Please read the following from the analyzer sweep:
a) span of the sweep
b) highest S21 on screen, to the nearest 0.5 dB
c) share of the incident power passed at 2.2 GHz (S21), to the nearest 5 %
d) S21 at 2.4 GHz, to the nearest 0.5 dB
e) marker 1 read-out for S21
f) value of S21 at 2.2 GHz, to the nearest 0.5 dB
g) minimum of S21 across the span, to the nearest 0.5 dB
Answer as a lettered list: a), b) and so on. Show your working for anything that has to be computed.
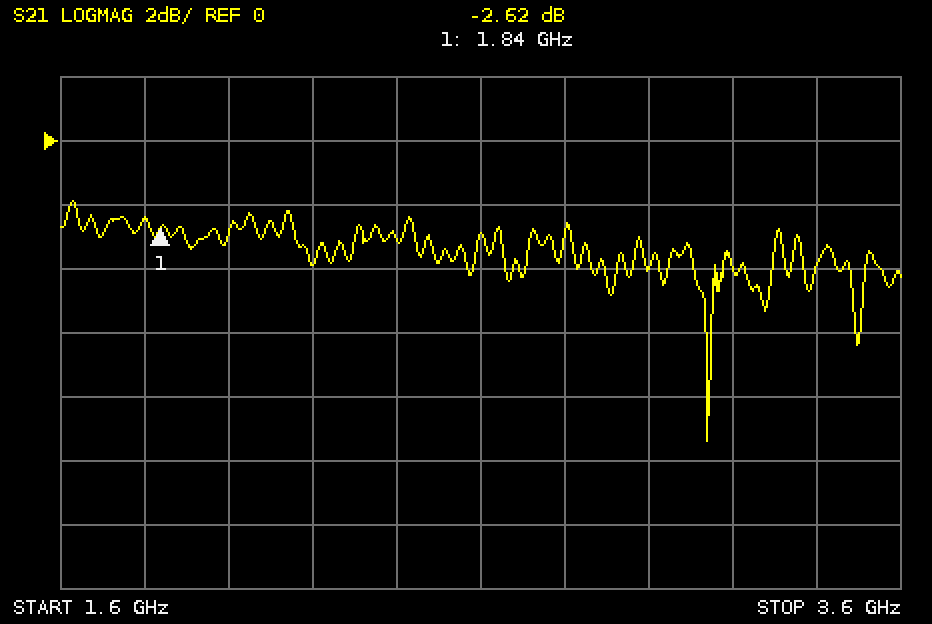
a) 2 GHz
b) -2.0 dB
c) 10^(-4/10) ≈ 40 %
d) -3.0 dB
e) -2.62 dB
f) -4.0 dB
g) -9.5 dB
